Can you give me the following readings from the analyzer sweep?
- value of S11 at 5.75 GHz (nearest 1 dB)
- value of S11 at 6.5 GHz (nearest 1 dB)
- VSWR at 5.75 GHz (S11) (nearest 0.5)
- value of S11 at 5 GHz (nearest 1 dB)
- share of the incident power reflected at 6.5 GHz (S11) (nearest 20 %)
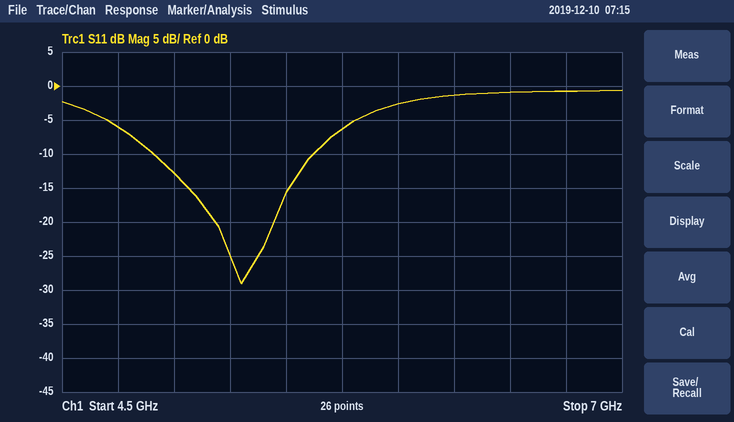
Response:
-6 dB
-1 dB
3.0
-13 dB
80 %
